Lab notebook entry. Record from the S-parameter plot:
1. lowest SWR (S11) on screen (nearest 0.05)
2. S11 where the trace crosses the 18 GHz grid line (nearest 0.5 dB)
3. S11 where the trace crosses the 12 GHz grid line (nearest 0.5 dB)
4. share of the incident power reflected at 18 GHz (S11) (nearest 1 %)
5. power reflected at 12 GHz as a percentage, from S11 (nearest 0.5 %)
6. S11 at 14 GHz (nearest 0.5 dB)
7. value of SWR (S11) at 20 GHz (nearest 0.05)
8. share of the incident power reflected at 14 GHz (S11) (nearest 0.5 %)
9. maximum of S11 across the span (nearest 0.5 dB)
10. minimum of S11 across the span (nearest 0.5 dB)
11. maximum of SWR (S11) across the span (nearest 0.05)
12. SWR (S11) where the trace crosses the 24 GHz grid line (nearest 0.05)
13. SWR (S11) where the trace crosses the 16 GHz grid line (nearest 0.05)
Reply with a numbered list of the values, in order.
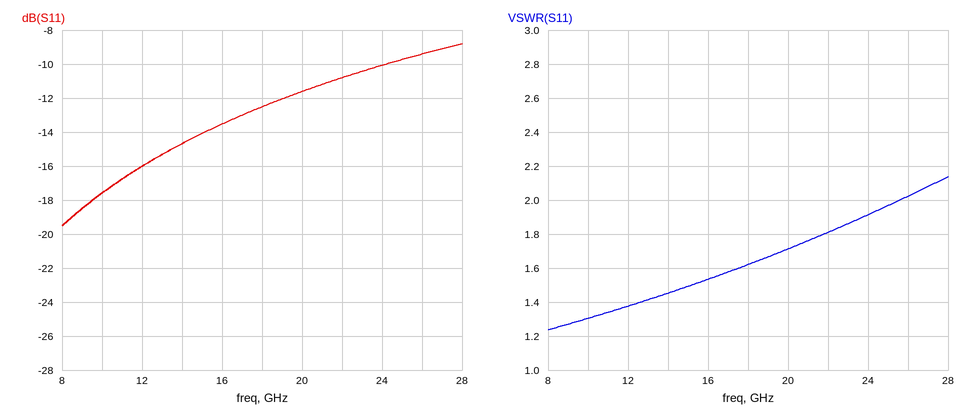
1. 1.25
2. -12.5 dB
3. -16.0 dB
4. 6 %
5. 2.5 %
6. -14.5 dB
7. 1.70
8. 3.5 %
9. -9.0 dB
10. -19.5 dB
11. 2.15
12. 1.90
13. 1.55
